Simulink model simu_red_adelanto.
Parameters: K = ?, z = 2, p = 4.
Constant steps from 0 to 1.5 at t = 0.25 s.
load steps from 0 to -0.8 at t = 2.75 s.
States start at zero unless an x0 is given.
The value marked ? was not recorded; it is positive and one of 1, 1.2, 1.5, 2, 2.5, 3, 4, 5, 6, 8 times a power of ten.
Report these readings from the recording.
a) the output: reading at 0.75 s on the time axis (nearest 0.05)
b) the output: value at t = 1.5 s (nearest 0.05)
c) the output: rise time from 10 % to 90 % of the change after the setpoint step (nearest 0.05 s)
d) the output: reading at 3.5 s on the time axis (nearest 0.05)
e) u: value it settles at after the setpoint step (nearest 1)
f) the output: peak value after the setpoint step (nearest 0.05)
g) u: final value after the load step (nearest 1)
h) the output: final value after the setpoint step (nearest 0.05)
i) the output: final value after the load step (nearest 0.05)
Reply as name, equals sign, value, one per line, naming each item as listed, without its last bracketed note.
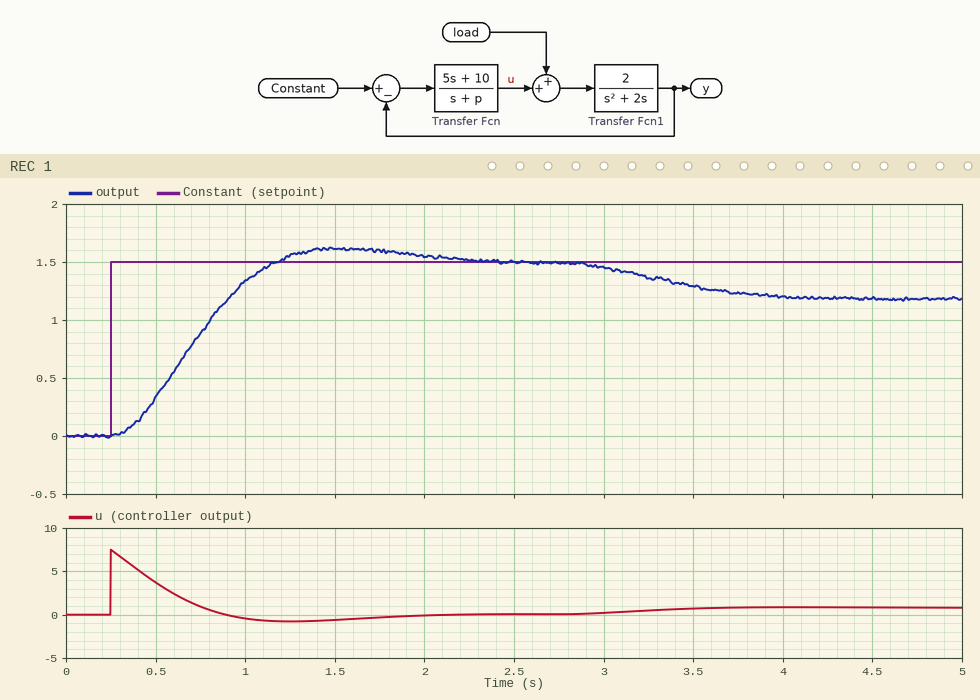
the output: reading at 0.75 s on the time axis = 0.90
the output: value at t = 1.5 s = 1.60
the output: rise time from 10 % to 90 % of the change after the setpoint step = 0.60 s
the output: reading at 3.5 s on the time axis = 1.30
u: value it settles at after the setpoint step = 0
the output: peak value after the setpoint step = 1.60
u: final value after the load step = 1
the output: final value after the setpoint step = 1.50
the output: final value after the load step = 1.20
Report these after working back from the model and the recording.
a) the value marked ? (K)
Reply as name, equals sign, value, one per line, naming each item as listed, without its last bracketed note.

the value marked ? = 5
